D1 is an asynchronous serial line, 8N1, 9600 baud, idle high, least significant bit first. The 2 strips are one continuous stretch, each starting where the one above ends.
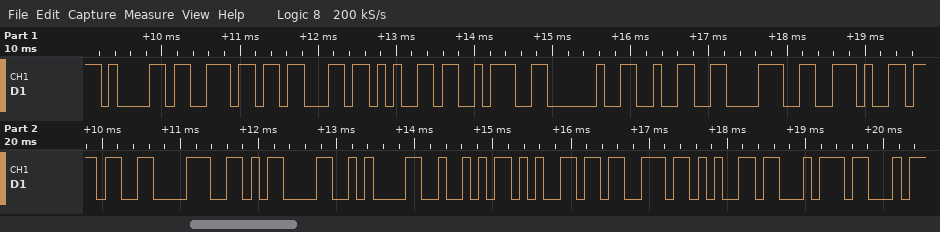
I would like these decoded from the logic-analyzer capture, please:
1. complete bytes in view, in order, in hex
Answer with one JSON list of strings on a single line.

["0x61 0x6E 0x63 0x65 0x3A 0x20 0x32 0x38 0x2E 0x37 0x38 0x0D 0x0A 0x52 0x65 0x73 0x65 0x74"]
